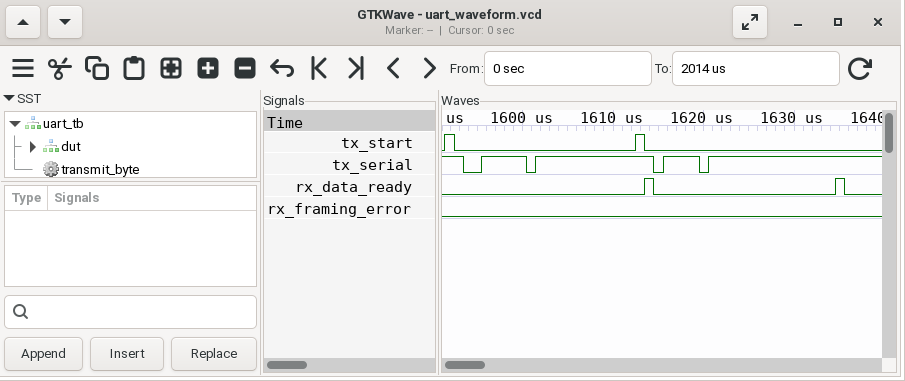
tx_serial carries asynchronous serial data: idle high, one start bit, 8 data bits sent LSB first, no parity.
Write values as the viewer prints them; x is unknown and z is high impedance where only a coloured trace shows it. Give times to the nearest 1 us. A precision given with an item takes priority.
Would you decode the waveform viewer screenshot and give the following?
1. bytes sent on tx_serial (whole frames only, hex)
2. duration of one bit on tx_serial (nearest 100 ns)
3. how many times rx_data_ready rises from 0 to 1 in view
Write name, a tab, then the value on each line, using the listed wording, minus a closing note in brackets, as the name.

bytes sent on tx_serial	BE, EF
duration of one bit on tx_serial	1000 ns
how many times rx_data_ready rises from 0 to 1 in view	2
